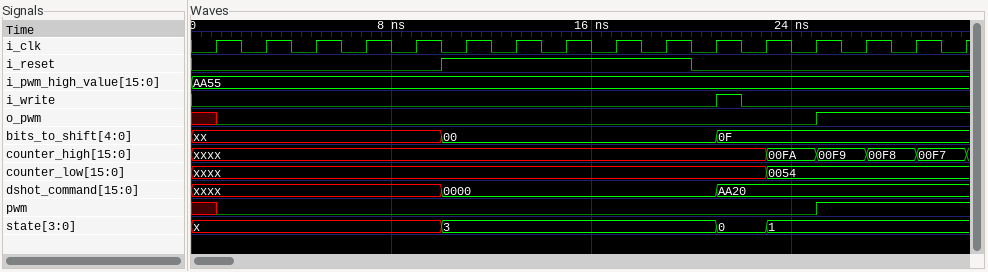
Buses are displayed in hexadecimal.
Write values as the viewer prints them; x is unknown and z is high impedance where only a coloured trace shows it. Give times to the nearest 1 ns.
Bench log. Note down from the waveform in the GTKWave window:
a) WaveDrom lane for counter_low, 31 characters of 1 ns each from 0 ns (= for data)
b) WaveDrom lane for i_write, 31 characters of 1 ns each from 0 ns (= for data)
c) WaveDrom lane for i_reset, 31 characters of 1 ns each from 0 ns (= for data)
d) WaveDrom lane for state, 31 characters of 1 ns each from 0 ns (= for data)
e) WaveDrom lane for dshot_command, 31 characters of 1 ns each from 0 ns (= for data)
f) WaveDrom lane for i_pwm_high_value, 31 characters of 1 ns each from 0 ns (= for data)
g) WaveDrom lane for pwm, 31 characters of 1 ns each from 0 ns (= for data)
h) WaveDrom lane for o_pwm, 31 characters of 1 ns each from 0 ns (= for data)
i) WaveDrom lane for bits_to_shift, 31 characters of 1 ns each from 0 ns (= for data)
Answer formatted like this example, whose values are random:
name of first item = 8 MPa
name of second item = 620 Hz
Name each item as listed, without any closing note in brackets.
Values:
WaveDrom lane for counter_low, 31 characters of 1 ns each from 0 ns = {name: 'counter_low', wave: 'x......................=.......', data: '0054'}
WaveDrom lane for i_write, 31 characters of 1 ns each from 0 ns = {name: 'i_write', wave: '0....................10........'}
WaveDrom lane for i_reset, 31 characters of 1 ns each from 0 ns = {name: 'i_reset', wave: '0.........1.........0..........'}
WaveDrom lane for state, 31 characters of 1 ns each from 0 ns = {name: 'state', wave: 'x.........=..........=.=.......', data: '3 0 1'}
WaveDrom lane for dshot_command, 31 characters of 1 ns each from 0 ns = {name: 'dshot_command', wave: 'x.........=..........=.........', data: '0000 AA20'}
WaveDrom lane for i_pwm_high_value, 31 characters of 1 ns each from 0 ns = {name: 'i_pwm_high_value', wave: '=..............................', data: 'AA55'}
WaveDrom lane for pwm, 31 characters of 1 ns each from 0 ns = {name: 'pwm', wave: 'x0.......................1.....'}
WaveDrom lane for o_pwm, 31 characters of 1 ns each from 0 ns = {name: 'o_pwm', wave: 'x0.......................1.....'}
WaveDrom lane for bits_to_shift, 31 characters of 1 ns each from 0 ns = {name: 'bits_to_shift', wave: 'x.........=..........=.........', data: '00 0F'}
